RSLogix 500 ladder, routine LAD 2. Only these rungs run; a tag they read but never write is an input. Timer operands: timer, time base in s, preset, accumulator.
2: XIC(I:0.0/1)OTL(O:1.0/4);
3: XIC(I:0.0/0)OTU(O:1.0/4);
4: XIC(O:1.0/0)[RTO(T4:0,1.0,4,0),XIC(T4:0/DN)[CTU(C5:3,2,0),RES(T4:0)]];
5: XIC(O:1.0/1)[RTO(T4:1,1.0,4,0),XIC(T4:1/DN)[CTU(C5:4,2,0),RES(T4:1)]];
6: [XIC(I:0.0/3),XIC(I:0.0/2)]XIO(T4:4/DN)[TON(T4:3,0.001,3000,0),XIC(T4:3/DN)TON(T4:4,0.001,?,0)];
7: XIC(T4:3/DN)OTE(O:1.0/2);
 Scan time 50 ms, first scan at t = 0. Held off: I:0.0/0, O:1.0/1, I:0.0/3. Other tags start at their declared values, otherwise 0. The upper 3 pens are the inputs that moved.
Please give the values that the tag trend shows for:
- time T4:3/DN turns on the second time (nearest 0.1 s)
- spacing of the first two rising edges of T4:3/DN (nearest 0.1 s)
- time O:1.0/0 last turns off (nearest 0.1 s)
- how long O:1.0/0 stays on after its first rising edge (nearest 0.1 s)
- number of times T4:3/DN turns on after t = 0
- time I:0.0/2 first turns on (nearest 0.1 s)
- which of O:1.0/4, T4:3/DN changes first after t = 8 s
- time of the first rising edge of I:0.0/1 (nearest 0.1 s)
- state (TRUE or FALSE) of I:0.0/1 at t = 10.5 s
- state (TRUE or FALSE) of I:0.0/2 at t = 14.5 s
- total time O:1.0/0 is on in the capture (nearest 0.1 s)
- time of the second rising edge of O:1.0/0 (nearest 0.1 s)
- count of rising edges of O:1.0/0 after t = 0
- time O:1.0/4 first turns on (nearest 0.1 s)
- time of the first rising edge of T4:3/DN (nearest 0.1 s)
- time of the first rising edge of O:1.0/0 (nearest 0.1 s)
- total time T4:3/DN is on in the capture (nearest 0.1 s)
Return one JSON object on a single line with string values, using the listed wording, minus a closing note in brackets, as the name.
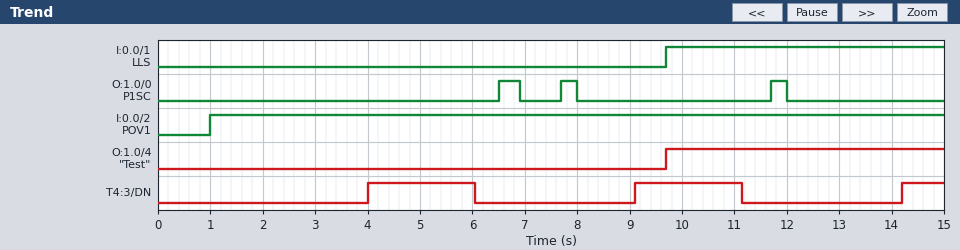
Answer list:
{"time T4:3/DN turns on the second time": "9.1 s", "spacing of the first two rising edges of T4:3/DN": "5.1 s", "time O:1.0/0 last turns off": "12.0 s", "how long O:1.0/0 stays on after its first rising edge": "0.4 s", "number of times T4:3/DN turns on after t = 0": "3", "time I:0.0/2 first turns on": "1.0 s", "which of O:1.0/4, T4:3/DN changes first after t = 8 s": "T4:3/DN", "time of the first rising edge of I:0.0/1": "9.7 s", "state (TRUE or FALSE) of I:0.0/1 at t = 10.5 s": "TRUE", "state (TRUE or FALSE) of I:0.0/2 at t = 14.5 s": "TRUE", "total time O:1.0/0 is on in the capture": "1.0 s", "time of the second rising edge of O:1.0/0": "7.7 s", "count of rising edges of O:1.0/0 after t = 0": "3", "time O:1.0/4 first turns on": "9.7 s", "time of the first rising edge of T4:3/DN": "4.0 s", "time of the first rising edge of O:1.0/0": "6.5 s", "total time T4:3/DN is on in the capture": "4.9 s"}
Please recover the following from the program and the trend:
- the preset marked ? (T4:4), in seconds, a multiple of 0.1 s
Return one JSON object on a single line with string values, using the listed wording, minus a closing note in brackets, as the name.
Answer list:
{"the preset marked ? (T4:4), in seconds, a multiple of 0.1 s": "2.0 s"}
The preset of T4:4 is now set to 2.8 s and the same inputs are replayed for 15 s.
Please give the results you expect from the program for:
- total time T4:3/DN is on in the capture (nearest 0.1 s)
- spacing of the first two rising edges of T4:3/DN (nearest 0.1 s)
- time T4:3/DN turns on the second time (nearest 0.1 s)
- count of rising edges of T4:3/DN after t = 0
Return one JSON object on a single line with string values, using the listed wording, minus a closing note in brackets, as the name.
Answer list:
{"total time T4:3/DN is on in the capture": "5.7 s", "spacing of the first two rising edges of T4:3/DN": "5.9 s", "time T4:3/DN turns on the second time": "9.9 s", "count of rising edges of T4:3/DN after t = 0": "2"}
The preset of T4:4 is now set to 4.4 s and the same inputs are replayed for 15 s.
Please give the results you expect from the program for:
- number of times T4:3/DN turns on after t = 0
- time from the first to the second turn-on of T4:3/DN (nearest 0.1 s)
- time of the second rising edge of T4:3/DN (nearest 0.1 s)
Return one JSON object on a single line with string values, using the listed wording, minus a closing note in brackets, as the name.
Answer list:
{"number of times T4:3/DN turns on after t = 0": "2", "time from the first to the second turn-on of T4:3/DN": "7.5 s", "time of the second rising edge of T4:3/DN": "11.5 s"}
